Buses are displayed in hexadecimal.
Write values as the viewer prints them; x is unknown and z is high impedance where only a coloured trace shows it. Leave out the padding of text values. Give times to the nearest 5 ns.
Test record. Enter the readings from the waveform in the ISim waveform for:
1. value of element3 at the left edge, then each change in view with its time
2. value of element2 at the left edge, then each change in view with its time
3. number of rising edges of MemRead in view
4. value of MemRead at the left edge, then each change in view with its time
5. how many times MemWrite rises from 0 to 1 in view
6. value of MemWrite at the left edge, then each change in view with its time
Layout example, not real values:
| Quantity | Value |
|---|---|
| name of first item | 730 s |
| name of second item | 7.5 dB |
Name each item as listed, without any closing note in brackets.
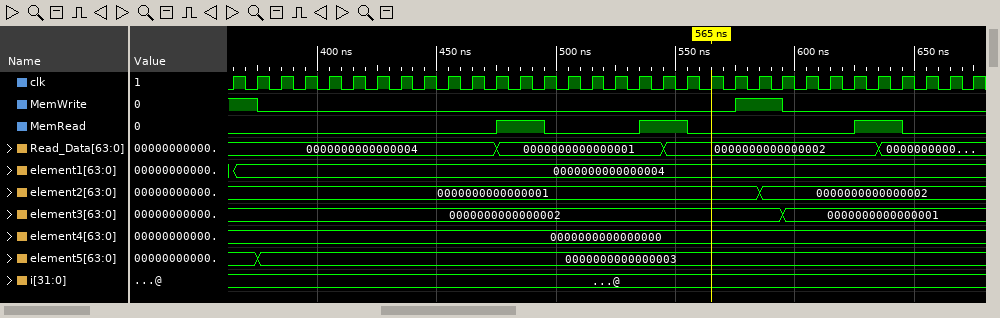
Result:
| Quantity | Value |
|---|---|
| value of element3 at the left edge, then each change in view with its time | 0000000000000002, 0000000000000001 at 595 ns |
| value of element2 at the left edge, then each change in view with its time | 0000000000000001, 0000000000000002 at 585 ns |
| number of rising edges of MemRead in view | 3 |
| value of MemRead at the left edge, then each change in view with its time | 0, 1 at 475 ns, 0 at 495 ns, 1 at 535 ns, 0 at 555 ns, 1 at 625 ns, 0 at 645 ns |
| how many times MemWrite rises from 0 to 1 in view | 1 |
| value of MemWrite at the left edge, then each change in view with its time | 1, 0 at 375 ns, 1 at 575 ns, 0 at 595 ns |
